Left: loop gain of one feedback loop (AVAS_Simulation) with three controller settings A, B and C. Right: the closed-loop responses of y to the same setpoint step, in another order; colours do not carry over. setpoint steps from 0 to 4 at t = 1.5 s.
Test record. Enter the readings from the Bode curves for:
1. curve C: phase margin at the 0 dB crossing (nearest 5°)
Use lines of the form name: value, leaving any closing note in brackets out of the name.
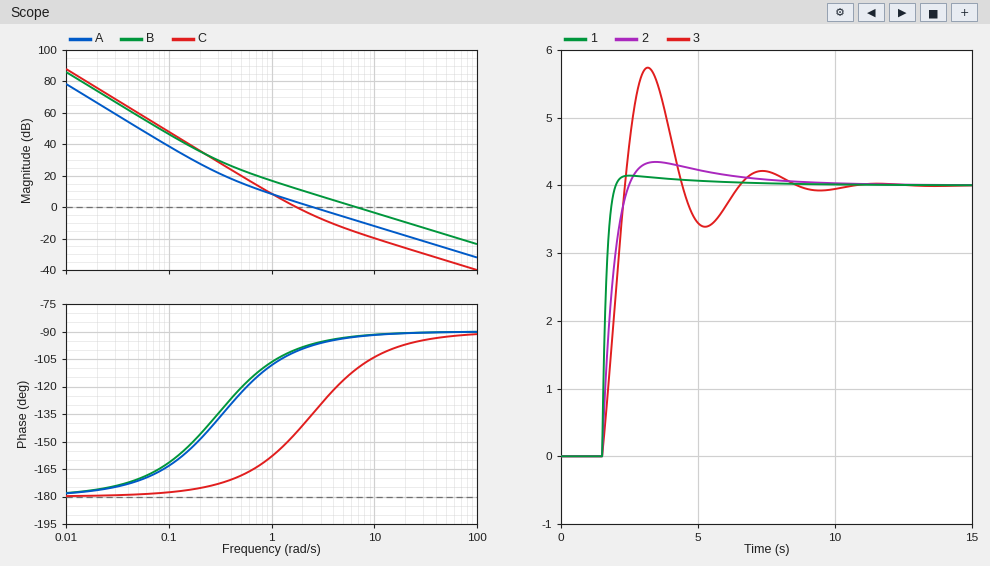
curve C: phase margin at the 0 dB crossing: 35°
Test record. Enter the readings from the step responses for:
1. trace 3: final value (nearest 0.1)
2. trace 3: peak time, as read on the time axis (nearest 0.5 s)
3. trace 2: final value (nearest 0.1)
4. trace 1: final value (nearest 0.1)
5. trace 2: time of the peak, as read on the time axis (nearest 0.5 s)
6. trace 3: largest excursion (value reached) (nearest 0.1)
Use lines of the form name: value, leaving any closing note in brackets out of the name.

trace 3: final value: 4.0
trace 3: peak time, as read on the time axis: 3.0 s
trace 2: final value: 4.0
trace 1: final value: 4.0
trace 2: time of the peak, as read on the time axis: 3.5 s
trace 3: largest excursion (value reached): 5.7
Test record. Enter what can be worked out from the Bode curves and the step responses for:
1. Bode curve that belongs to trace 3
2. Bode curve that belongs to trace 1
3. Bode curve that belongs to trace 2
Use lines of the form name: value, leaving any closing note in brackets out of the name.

Bode curve that belongs to trace 3: C
Bode curve that belongs to trace 1: B
Bode curve that belongs to trace 2: A
